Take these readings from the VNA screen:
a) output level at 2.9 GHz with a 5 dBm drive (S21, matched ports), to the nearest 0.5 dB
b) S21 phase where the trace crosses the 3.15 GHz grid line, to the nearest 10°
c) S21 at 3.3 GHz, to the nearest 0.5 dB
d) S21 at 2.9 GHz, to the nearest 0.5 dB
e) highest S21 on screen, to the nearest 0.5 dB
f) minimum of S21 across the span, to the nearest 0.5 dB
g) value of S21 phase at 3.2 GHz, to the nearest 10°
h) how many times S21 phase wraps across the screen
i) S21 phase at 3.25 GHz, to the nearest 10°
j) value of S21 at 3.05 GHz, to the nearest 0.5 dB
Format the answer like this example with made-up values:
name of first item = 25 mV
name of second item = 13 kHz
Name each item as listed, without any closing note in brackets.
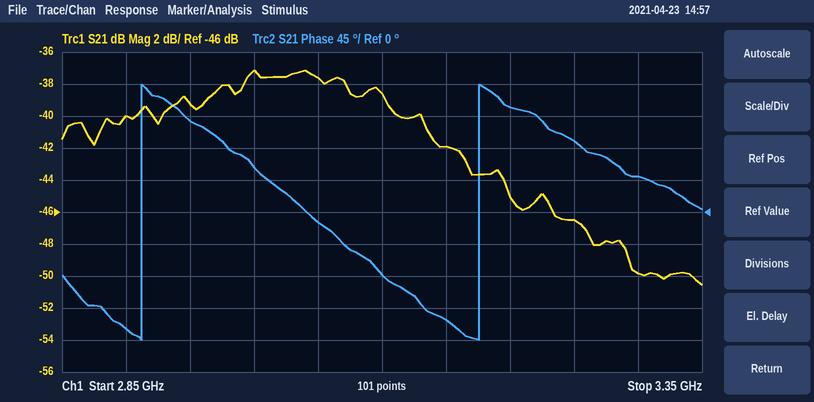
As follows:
output level at 2.9 GHz with a 5 dBm drive (S21, matched ports), to the nearest 0.5 dB = -35.0 dBm
S21 phase where the trace crosses the 3.15 GHz grid line, to the nearest 10° = -150°
S21 at 3.3 GHz, to the nearest 0.5 dB = -50.0 dB
S21 at 2.9 GHz, to the nearest 0.5 dB = -40.0 dB
highest S21 on screen, to the nearest 0.5 dB = -37.0 dB
minimum of S21 across the span, to the nearest 0.5 dB = -50.5 dB
value of S21 phase at 3.2 GHz, to the nearest 10° = 150°
how many times S21 phase wraps across the screen = 2
S21 phase at 3.25 GHz, to the nearest 10° = 100°
value of S21 at 3.05 GHz, to the nearest 0.5 dB = -37.5 dB
